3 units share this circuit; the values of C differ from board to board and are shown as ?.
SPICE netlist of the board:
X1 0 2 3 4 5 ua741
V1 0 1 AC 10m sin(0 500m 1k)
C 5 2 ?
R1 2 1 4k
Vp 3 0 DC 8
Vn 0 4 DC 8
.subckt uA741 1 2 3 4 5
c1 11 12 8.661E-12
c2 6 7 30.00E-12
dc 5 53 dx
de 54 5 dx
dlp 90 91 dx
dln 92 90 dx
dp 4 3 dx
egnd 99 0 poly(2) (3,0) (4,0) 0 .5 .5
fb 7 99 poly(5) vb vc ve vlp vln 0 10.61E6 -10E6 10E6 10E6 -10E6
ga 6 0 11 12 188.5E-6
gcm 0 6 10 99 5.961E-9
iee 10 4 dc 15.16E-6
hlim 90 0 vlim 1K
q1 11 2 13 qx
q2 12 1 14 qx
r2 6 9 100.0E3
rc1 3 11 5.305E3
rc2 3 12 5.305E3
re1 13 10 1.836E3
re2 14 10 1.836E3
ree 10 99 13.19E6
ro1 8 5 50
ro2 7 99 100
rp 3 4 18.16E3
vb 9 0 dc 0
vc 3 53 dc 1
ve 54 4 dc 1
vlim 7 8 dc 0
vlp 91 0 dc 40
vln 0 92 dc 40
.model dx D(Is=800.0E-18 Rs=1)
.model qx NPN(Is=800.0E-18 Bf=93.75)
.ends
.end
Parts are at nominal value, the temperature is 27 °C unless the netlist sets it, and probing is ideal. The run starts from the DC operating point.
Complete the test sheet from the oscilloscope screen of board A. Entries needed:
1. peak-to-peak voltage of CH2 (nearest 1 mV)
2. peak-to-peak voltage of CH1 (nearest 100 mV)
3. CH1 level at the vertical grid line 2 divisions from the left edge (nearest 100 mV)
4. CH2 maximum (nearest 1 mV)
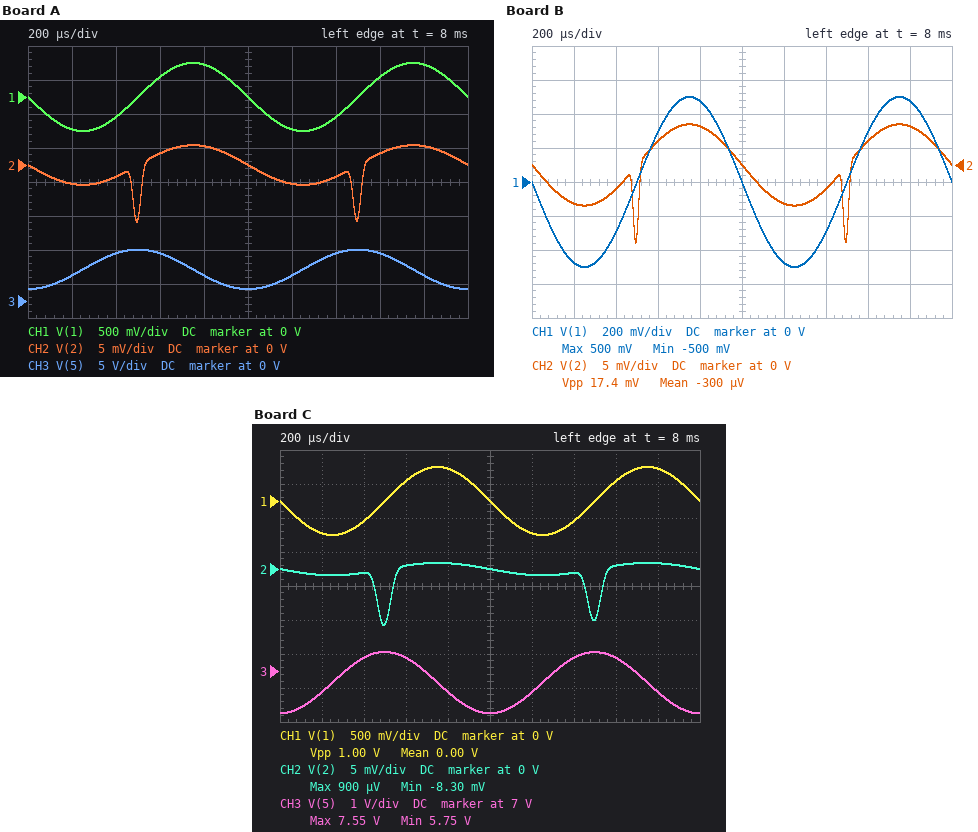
11 mV
1.0 V
-300 mV
3 mV
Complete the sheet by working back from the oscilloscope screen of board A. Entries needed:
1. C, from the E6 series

6.8 nF
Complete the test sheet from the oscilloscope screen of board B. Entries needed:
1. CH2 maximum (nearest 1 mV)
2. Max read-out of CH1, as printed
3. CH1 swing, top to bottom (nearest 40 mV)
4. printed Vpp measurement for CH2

6 mV
500 mV
1.00 V
17.4 mV
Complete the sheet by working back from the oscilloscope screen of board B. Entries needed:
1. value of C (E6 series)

3.3 nF
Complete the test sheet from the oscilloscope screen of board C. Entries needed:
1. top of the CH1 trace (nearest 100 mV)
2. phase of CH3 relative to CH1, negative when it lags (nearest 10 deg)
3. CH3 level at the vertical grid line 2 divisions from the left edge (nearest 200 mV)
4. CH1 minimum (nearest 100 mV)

500 mV
90 deg
7.4 V
-500 mV
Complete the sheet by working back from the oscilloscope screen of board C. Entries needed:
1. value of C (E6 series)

22 nF
